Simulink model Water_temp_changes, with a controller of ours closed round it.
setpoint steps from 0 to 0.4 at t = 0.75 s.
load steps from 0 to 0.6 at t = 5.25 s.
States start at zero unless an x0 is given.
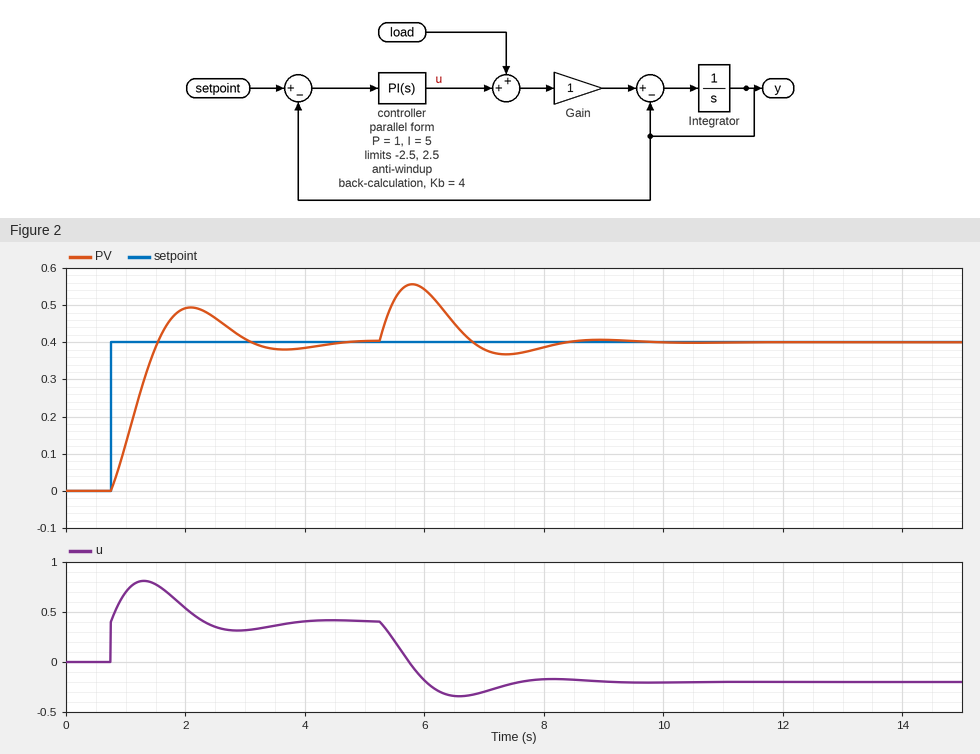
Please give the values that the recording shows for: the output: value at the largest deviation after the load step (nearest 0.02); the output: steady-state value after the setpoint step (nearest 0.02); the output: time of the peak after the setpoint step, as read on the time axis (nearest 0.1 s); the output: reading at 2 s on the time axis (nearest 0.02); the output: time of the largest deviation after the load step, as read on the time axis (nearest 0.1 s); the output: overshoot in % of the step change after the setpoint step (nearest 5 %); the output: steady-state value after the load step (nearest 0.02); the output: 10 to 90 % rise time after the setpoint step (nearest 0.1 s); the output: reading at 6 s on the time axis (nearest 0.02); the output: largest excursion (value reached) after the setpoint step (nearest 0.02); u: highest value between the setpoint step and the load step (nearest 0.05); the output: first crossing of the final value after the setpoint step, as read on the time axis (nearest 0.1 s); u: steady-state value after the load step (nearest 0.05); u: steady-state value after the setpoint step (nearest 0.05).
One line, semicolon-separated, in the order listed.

0.56; 0.40; 2.1 s; 0.50; 5.8 s; 25 %; 0.40; 0.6 s; 0.54; 0.50; 0.80; 1.5 s; -0.20; 0.40
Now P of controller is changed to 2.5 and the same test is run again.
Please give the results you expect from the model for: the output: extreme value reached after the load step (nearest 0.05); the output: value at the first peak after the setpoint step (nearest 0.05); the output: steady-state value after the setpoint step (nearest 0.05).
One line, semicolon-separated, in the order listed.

0.50; 0.45; 0.40
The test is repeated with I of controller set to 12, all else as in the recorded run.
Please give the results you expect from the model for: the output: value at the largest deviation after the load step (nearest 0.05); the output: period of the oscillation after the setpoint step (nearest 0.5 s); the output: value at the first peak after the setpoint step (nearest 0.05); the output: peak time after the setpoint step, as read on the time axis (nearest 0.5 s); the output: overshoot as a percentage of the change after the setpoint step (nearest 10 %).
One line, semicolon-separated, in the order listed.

0.50; 2.0 s; 0.55; 1.5 s; 40 %
